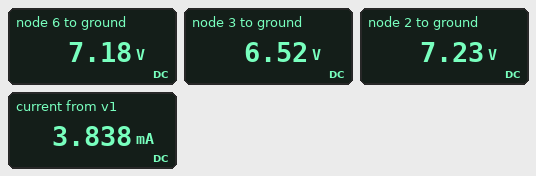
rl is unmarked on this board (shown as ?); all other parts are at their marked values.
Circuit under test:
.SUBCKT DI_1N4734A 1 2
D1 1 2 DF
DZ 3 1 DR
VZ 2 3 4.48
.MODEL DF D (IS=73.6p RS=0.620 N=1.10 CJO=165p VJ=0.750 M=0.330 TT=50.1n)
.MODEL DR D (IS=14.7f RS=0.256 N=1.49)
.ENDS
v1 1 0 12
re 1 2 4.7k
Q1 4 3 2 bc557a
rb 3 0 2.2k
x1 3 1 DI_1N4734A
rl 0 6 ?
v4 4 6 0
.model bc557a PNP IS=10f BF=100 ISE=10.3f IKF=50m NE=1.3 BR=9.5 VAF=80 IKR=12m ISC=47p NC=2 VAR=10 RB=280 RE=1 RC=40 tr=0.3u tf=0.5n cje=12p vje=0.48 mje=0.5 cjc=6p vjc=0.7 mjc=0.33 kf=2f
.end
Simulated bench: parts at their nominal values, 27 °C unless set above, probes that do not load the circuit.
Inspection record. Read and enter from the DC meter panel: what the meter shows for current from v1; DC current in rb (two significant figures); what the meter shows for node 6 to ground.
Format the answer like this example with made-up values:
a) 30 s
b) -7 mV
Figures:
a) 3.838 mA
b) 3.0 mA
c) 7.18 V
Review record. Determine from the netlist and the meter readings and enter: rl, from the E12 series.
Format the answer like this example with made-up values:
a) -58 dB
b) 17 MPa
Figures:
a) 8.2 kΩ
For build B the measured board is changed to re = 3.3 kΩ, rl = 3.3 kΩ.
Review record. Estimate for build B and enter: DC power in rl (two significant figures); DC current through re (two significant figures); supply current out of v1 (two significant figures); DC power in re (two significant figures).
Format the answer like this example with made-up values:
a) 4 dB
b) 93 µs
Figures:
a) 6.8 mW
b) 1.5 mA
c) 4.4 mA
d) 7.0 mW
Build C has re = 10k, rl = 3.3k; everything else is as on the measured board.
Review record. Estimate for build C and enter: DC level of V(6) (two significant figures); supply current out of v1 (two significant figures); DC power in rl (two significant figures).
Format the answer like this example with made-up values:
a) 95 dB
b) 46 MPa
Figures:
a) 1.6 V
b) 3.4 mA
c) 750 µW
